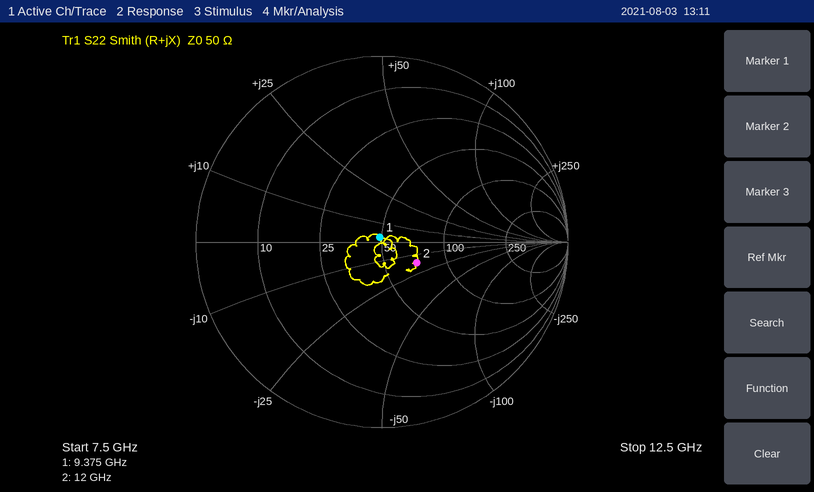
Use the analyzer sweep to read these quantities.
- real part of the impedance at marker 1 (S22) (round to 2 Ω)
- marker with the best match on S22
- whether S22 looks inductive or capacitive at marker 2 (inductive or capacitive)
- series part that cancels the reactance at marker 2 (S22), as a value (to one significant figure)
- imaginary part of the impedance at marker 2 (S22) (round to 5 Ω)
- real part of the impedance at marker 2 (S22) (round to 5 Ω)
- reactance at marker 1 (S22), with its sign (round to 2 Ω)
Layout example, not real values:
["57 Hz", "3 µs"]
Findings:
["48 Ω", "marker 1", "capacitive", "200 pH", "-15 Ω", "70 Ω", "+2 Ω"]
